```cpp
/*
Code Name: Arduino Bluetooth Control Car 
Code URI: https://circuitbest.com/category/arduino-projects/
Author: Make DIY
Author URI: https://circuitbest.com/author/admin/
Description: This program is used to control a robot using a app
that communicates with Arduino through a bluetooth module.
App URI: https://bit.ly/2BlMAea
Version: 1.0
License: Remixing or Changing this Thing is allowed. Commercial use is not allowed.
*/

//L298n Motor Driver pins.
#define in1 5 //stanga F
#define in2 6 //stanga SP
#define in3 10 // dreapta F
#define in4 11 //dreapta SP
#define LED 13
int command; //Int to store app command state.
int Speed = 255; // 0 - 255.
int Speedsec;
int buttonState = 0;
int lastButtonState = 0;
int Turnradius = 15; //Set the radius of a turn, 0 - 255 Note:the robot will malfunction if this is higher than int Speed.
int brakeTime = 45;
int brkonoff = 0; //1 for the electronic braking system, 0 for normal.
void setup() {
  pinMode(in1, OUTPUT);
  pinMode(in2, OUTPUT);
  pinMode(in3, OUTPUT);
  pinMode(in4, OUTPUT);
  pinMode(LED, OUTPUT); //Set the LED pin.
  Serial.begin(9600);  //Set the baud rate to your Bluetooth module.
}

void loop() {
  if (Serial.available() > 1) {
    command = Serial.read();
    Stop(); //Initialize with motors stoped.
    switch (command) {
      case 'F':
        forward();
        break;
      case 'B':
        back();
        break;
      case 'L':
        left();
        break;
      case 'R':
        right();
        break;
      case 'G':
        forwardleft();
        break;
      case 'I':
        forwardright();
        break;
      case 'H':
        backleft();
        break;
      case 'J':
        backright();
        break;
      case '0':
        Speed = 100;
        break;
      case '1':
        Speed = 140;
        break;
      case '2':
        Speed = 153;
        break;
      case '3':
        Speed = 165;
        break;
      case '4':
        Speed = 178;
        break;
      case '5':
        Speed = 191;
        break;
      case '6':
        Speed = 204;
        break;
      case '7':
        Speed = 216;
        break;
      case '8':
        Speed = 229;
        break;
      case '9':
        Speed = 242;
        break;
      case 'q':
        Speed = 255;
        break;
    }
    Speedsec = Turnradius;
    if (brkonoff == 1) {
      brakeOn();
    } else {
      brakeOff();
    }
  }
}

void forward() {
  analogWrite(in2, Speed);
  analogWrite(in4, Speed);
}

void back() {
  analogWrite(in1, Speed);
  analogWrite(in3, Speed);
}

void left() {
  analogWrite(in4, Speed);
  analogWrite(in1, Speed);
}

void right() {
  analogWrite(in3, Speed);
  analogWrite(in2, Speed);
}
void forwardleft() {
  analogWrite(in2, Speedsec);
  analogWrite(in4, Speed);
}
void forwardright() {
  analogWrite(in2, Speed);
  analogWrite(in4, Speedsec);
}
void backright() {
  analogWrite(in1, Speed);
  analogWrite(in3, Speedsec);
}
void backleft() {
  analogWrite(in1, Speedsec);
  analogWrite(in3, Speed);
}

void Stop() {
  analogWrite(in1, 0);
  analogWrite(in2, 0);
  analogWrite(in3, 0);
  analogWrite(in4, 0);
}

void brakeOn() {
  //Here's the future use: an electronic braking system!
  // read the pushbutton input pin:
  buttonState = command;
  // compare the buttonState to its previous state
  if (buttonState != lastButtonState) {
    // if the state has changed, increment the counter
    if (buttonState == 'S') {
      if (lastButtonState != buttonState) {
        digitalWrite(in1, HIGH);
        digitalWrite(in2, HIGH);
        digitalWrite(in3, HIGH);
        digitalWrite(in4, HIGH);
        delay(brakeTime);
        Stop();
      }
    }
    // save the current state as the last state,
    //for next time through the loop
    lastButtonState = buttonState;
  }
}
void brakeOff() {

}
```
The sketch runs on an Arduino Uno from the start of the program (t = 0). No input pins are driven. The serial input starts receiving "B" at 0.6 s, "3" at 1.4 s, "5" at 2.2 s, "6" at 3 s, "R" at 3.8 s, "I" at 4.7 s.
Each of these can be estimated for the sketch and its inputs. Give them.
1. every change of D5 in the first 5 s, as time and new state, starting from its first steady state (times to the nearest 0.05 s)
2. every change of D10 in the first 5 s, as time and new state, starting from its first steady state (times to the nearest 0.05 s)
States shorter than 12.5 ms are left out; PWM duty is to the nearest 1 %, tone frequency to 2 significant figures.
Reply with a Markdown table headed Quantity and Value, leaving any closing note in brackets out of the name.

| Quantity | Value |
|---|---|
| every change of D5 in the first 5 s, as time and new state, starting from its first steady state | 0 s low; 1.4 s high; 2.2 s low |
| every change of D10 in the first 5 s, as time and new state, starting from its first steady state | 0 s low; 1.4 s high; 2.2 s low; 4.7 s PWM 80 % |
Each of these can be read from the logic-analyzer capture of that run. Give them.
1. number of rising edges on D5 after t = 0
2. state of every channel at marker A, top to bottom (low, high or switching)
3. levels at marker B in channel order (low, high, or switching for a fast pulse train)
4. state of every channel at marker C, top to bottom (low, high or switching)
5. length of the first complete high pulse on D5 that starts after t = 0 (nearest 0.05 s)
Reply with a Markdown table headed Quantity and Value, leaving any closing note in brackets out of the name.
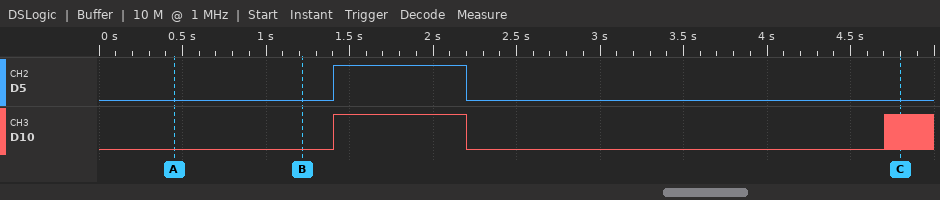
| Quantity | Value |
|---|---|
| number of rising edges on D5 after t = 0 | 1 |
| state of every channel at marker A, top to bottom | D5 low, D10 low |
| levels at marker B in channel order | D5 low, D10 low |
| state of every channel at marker C, top to bottom | D5 low, D10 switching |
| length of the first complete high pulse on D5 that starts after t = 0 | 0.80 s |
